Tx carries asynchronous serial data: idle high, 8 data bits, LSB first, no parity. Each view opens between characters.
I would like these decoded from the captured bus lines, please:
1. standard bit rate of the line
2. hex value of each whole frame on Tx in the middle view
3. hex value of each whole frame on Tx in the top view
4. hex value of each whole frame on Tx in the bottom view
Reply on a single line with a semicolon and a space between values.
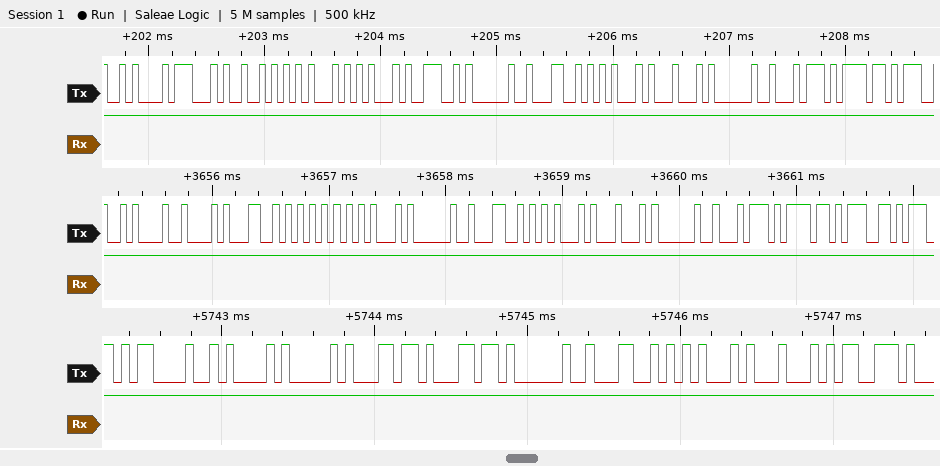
19200 baud; 0A, 42, 4C, 55, 45, 20, 4C, 45, 44, 20, 74, 6F, 67; 0A, 47, 52, 45, 45, 4E, 20, 4C, 45, 44, 20, 74, 6F; 0D, 0A, 41, 6C, 6C, 20, 4C, 45, 44, 73
